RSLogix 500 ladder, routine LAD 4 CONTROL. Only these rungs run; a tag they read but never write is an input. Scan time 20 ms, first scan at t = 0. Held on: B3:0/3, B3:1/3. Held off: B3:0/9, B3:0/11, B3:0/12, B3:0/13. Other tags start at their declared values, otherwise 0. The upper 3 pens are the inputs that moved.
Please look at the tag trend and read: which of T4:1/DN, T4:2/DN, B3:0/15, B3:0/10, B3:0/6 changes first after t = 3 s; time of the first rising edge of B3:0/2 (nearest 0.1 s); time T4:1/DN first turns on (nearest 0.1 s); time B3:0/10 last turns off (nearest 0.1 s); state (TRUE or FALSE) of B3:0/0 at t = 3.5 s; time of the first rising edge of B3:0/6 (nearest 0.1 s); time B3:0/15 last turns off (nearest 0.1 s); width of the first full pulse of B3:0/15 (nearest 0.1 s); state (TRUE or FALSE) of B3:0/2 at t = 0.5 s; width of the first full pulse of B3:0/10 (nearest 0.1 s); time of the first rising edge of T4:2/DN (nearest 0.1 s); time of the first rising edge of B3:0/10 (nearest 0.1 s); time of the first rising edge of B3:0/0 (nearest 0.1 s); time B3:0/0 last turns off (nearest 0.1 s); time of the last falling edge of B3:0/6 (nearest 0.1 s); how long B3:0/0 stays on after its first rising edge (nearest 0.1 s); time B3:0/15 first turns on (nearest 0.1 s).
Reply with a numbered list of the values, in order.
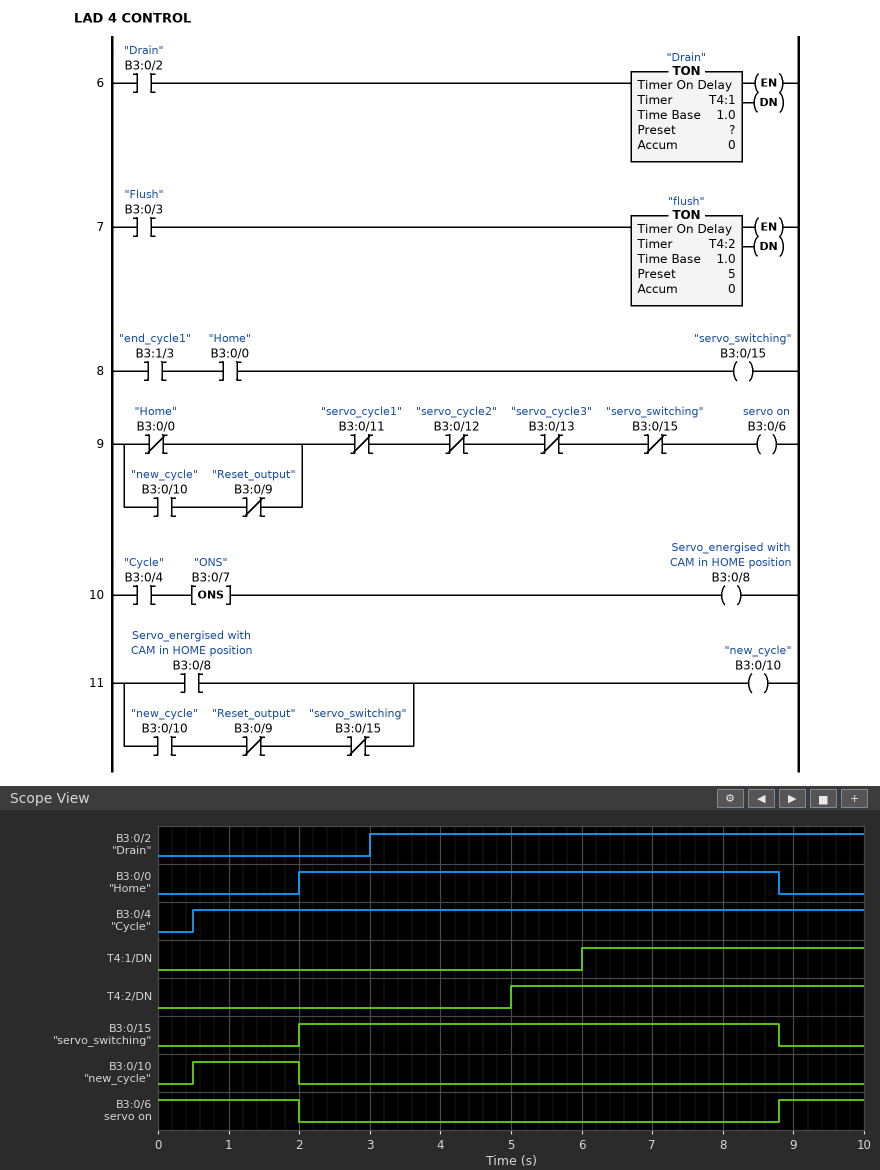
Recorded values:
1. T4:2/DN
2. 3.0 s
3. 6.0 s
4. 2.0 s
5. TRUE
6. 8.8 s
7. 8.8 s
8. 6.8 s
9. FALSE
10. 1.5 s
11. 5.0 s
12. 0.5 s
13. 2.0 s
14. 8.8 s
15. 2.0 s
16. 6.8 s
17. 2.0 s
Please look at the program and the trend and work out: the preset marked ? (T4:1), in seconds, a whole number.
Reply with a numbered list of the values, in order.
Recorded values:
1. 3 s
